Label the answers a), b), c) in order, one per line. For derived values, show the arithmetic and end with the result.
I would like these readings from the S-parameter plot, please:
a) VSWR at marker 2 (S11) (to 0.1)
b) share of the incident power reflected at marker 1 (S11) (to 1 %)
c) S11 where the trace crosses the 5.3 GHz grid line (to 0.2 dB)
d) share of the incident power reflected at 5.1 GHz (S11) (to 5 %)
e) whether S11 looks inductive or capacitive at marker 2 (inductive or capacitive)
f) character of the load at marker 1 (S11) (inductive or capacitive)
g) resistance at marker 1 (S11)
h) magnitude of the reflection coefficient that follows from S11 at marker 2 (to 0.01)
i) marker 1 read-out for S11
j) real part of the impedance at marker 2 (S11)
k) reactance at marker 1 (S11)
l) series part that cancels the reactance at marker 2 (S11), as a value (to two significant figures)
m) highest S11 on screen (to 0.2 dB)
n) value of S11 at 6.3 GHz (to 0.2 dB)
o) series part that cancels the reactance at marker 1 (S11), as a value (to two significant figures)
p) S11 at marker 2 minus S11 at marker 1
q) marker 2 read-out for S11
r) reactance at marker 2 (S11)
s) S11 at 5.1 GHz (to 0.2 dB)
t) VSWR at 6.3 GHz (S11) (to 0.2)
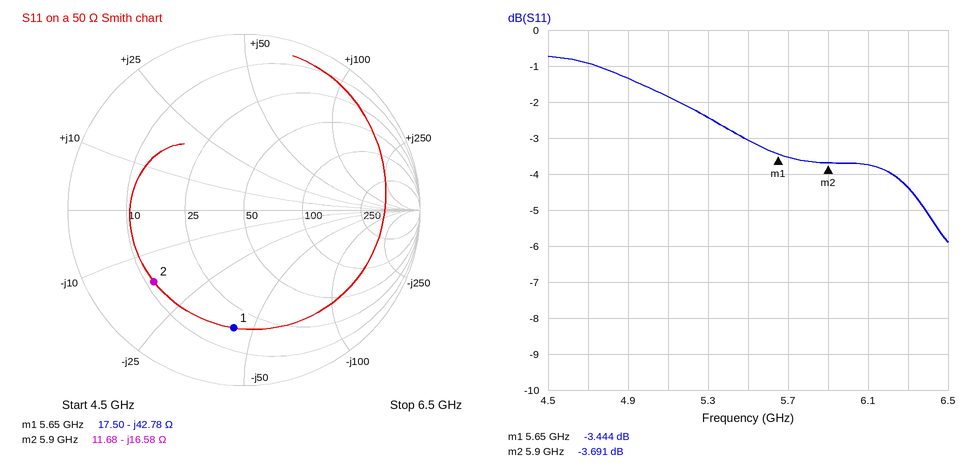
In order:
a) 4.8
b) 10^(-3.444/10) ≈ 45 %
c) -2.4 dB
d) 10^(-1.8/10) ≈ 66.1 %, so 65 % to the nearest 5 %
e) capacitive
f) capacitive
g) 17.50 Ω
h) 10^(-3.691/20) ≈ 0.65
i) -3.444 dB
j) 11.68 Ω
k) -42.78 Ω
l) L = 16.58 Ω/(2π × 5.9 GHz) ≈ 447 pH, so 450 pH to two significant figures
m) -0.8 dB
n) -4.4 dB
o) L = 42.78 Ω/(2π × 5.65 GHz) ≈ 1.2 nH
p) -3.691 − (-3.444) = -0.247 dB
q) -3.691 dB
r) -16.58 Ω
s) -1.8 dB
t) |Γ| = 10^(-4.4/20) = 0.6026; VSWR = (1 + 0.6026)/(1 − 0.6026) ≈ 4.0
